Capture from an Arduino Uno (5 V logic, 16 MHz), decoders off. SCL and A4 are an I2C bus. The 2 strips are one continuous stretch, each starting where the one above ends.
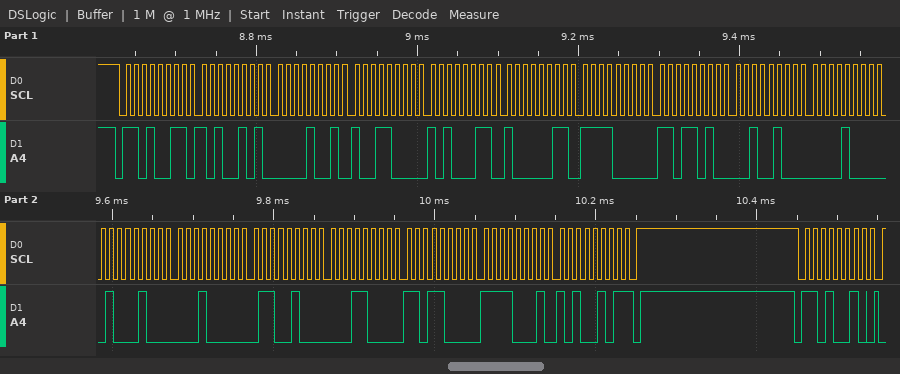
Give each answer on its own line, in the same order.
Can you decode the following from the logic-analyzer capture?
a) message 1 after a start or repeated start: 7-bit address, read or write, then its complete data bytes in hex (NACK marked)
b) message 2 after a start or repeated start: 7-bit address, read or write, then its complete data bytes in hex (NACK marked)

0x69 read: A5 09 98 A3 83 F0 DA 24 08 44 10 64 18 D8 F1 A5 NACK
0x69 write
